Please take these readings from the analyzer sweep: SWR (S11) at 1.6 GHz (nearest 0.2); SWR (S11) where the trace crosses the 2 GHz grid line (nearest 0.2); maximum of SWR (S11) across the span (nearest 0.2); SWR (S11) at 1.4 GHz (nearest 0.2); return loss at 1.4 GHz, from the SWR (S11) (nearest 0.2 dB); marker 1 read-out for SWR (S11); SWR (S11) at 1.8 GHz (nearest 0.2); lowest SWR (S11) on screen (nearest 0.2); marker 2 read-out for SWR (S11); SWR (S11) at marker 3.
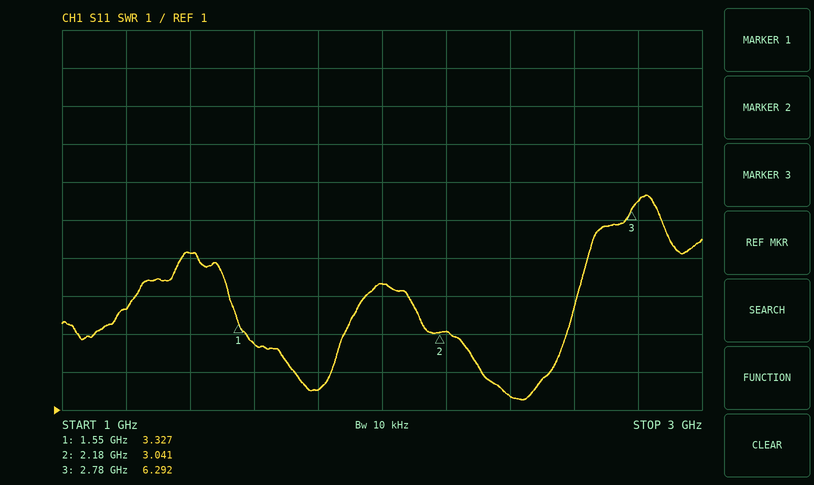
2.8
4.4
6.6
5.2
3.4 dB
3.327
1.6
1.2
3.041
6.292
